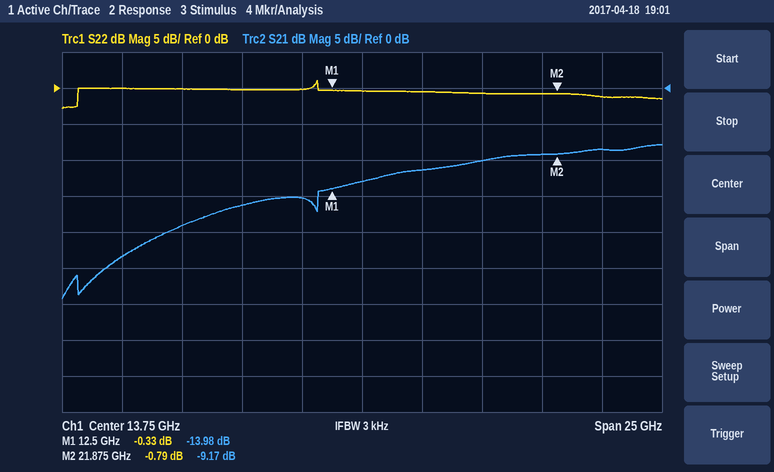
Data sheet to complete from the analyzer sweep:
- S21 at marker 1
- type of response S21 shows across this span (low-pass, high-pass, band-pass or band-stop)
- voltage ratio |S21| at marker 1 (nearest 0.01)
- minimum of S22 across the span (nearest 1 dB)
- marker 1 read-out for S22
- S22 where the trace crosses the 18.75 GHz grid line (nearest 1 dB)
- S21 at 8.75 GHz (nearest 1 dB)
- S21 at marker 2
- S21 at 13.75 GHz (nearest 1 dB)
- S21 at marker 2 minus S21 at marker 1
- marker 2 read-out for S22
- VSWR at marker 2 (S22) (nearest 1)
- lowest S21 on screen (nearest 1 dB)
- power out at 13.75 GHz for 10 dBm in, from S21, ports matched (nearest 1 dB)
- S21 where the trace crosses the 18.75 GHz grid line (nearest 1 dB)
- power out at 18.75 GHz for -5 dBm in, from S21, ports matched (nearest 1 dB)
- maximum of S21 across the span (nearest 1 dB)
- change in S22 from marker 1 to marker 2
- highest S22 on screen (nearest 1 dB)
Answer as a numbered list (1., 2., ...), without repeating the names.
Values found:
1. -13.98 dB
2. high-pass
3. 0.20
4. -3 dB
5. -0.33 dB
6. -1 dB
7. -16 dB
8. -9.17 dB
9. -13 dB
10. 4.81 dB
11. -0.79 dB
12. 22
13. -29 dB
14. -3 dBm
15. -10 dB
16. -15 dBm
17. -8 dB
18. -0.46 dB
19. 1 dB
